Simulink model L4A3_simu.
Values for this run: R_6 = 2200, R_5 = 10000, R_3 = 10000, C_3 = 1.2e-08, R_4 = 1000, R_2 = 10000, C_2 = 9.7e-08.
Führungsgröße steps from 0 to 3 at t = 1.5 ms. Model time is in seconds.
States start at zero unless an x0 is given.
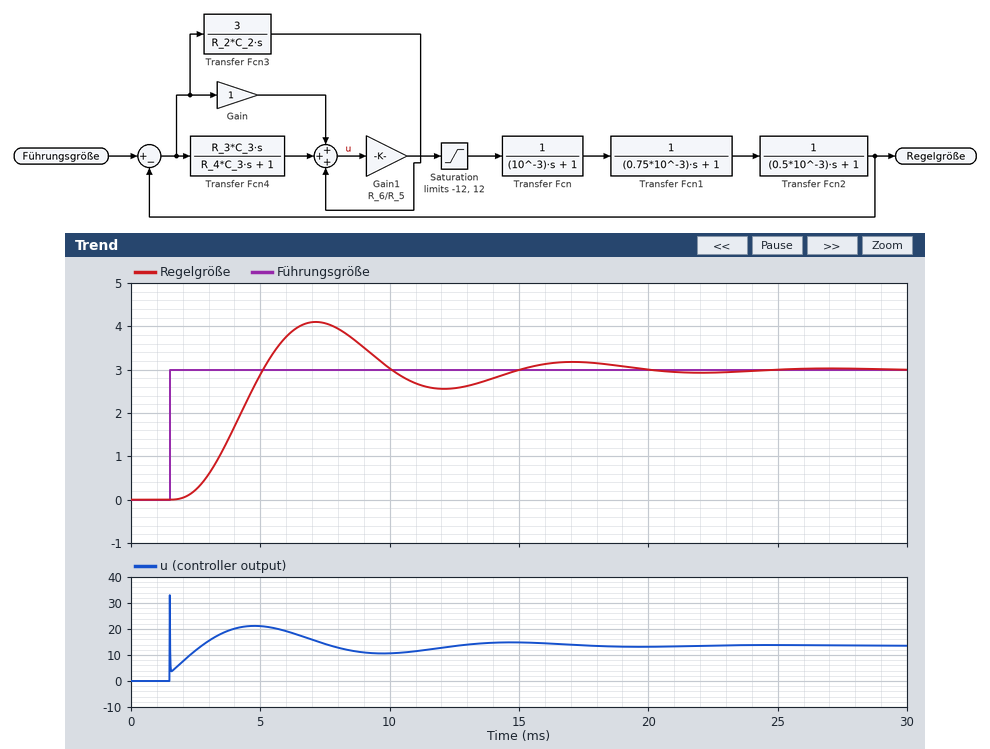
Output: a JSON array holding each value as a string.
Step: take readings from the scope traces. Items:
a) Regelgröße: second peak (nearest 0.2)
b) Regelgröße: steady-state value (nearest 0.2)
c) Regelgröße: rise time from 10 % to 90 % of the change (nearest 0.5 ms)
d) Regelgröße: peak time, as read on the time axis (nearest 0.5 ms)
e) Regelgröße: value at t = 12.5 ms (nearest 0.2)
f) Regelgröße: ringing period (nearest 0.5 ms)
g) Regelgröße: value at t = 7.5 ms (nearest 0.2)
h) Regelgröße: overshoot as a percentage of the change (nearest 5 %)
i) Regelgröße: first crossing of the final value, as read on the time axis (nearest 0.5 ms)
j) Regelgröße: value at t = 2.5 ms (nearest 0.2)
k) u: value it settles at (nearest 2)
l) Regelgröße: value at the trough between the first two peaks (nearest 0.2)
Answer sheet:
["3.2", "3.0", "2.0 ms", "7.0 ms", "2.6", "10.0 ms", "4.0", "35 %", "5.0 ms", "0.2", "14", "2.6"]
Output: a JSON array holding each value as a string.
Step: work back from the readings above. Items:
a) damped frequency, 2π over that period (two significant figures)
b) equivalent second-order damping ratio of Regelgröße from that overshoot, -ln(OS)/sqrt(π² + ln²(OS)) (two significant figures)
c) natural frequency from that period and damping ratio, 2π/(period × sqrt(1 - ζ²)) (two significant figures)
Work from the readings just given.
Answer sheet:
["0.63 rad/ms", "0.32", "0.66 rad/ms"]
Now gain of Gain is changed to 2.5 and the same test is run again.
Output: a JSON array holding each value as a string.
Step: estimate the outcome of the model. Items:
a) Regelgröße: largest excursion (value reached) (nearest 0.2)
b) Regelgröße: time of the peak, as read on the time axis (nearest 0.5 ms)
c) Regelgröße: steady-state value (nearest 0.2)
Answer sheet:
["3.6", "6.5 ms", "3.0"]
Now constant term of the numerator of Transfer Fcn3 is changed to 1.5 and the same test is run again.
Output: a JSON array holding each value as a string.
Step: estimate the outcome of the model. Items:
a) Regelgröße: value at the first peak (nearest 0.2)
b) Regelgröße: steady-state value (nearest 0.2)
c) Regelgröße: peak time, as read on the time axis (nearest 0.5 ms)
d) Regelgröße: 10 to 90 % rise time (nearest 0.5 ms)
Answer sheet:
["3.2", "3.0", "10.0 ms", "4.0 ms"]
